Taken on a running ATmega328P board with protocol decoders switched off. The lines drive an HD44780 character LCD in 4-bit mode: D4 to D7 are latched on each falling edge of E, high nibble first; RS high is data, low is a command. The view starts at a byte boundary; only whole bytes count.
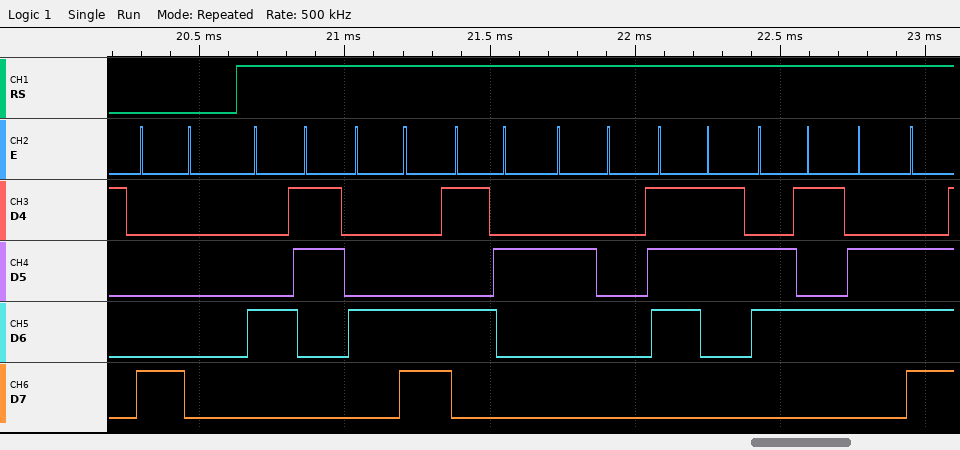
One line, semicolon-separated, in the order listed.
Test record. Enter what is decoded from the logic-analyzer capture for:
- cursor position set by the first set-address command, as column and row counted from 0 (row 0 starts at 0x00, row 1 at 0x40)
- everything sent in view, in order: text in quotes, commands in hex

column 0, row 0; 0x80 "CLR sen"
